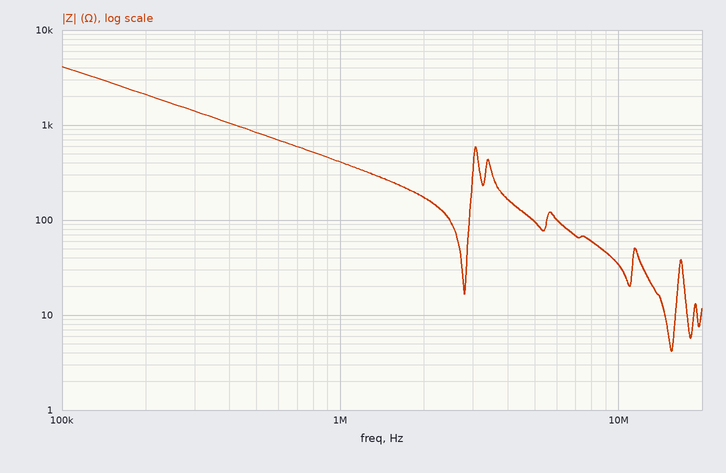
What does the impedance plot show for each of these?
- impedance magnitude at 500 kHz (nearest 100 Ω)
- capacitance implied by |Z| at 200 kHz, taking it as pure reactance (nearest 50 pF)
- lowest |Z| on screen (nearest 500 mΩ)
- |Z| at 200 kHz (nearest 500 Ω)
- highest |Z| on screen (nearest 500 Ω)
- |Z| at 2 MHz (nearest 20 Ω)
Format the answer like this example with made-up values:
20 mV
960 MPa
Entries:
800 Ω
400 pF
4.0 Ω
2.0 kΩ
4.0 kΩ
180 Ω
